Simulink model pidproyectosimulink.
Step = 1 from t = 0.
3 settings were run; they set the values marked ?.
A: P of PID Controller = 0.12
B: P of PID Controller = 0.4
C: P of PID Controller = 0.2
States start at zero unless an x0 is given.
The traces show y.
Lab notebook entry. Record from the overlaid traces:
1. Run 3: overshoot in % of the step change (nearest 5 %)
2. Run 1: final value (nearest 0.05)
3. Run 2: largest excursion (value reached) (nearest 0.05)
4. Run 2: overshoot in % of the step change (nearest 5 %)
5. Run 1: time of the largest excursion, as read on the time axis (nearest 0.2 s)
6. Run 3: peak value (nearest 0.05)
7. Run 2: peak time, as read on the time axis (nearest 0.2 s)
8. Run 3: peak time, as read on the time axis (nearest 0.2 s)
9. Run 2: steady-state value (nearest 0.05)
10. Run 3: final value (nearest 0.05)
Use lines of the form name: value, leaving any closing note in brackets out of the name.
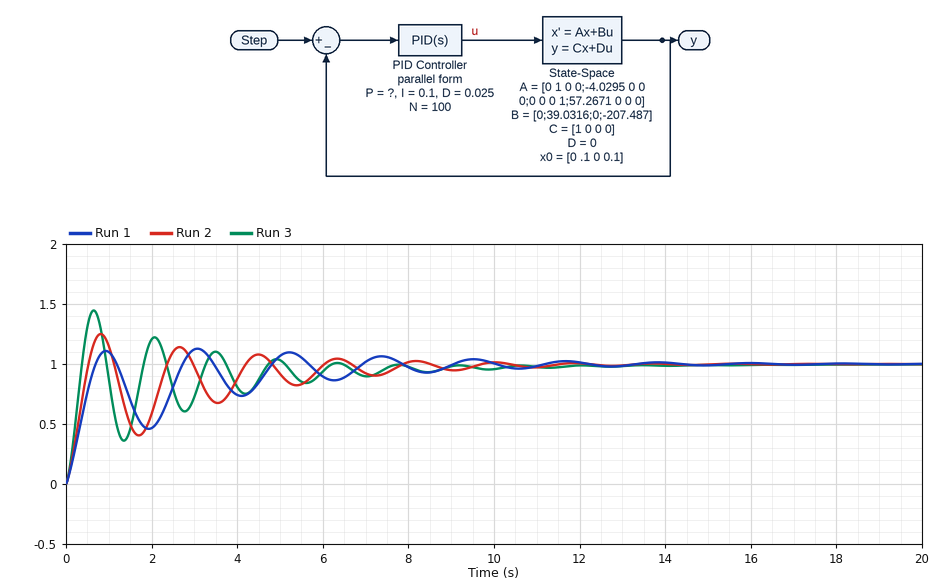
Run 3: overshoot in % of the step change: 45 %
Run 1: final value: 1.00
Run 2: largest excursion (value reached): 1.25
Run 2: overshoot in % of the step change: 25 %
Run 1: time of the largest excursion, as read on the time axis: 3.0 s
Run 3: peak value: 1.45
Run 2: peak time, as read on the time axis: 0.8 s
Run 3: peak time, as read on the time axis: 0.6 s
Run 2: steady-state value: 1.00
Run 3: final value: 1.00
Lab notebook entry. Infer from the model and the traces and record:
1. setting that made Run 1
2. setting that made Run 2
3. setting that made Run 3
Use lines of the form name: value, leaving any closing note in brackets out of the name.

setting that made Run 1: A
setting that made Run 2: C
setting that made Run 3: B
